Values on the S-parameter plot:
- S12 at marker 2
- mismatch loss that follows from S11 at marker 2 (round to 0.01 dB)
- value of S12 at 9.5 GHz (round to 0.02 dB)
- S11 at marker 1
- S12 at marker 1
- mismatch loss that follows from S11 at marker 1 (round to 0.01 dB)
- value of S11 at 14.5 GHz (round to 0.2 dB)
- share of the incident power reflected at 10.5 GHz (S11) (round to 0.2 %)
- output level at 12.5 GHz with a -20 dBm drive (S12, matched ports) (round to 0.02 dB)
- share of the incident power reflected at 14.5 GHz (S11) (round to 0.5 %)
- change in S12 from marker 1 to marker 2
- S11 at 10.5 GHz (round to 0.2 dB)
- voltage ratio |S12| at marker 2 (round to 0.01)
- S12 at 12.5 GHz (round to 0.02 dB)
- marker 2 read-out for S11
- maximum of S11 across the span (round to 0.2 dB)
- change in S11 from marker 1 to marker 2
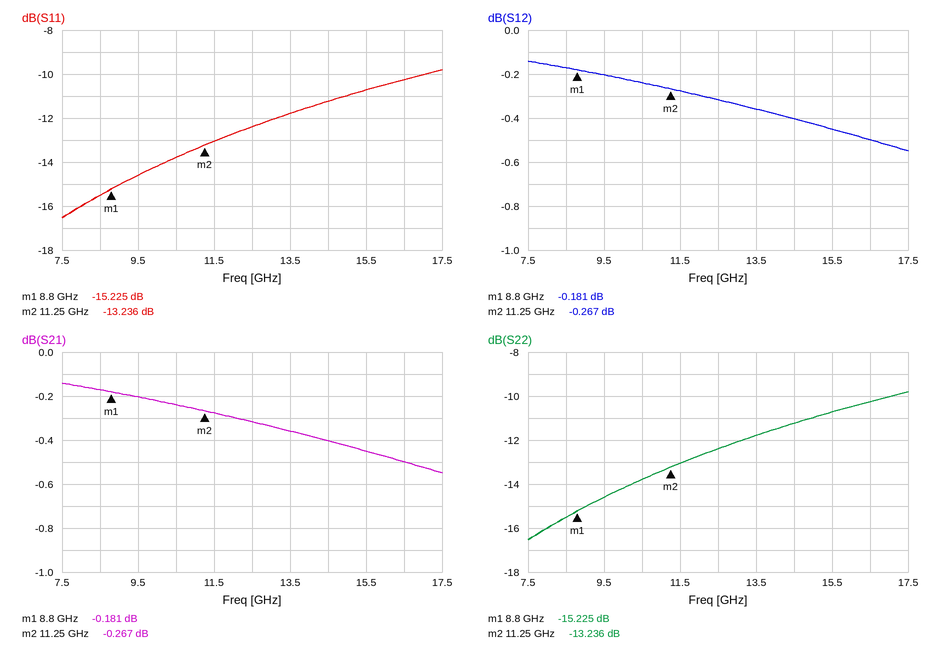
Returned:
-0.267 dB
0.21 dB
-0.20 dB
-15.225 dB
-0.181 dB
0.13 dB
-11.2 dB
4.2 %
-20.32 dBm
7.5 %
-0.086 dB
-13.8 dB
0.97
-0.32 dB
-13.236 dB
-9.8 dB
1.989 dB
